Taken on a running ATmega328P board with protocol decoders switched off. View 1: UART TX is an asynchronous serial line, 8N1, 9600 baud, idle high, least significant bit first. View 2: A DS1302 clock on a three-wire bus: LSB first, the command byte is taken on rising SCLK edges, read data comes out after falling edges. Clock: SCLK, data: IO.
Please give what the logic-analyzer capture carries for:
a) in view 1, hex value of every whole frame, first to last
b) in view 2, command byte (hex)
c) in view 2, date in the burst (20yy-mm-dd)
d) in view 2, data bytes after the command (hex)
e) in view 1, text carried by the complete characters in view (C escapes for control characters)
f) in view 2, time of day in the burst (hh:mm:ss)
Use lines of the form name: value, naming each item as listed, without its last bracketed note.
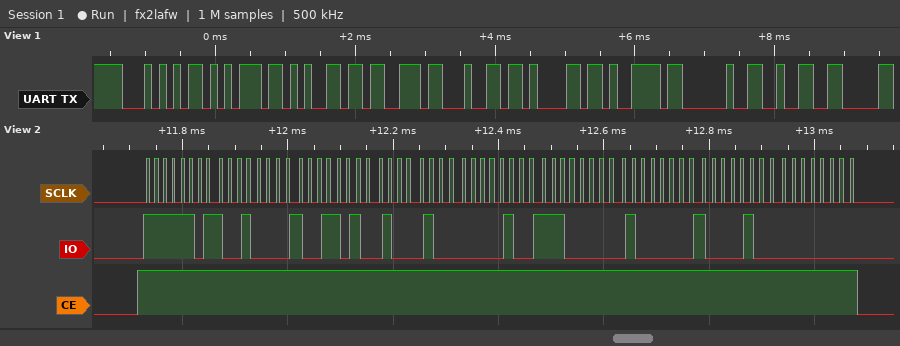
in view 1, hex value of every whole frame, first to last: 54 75 65 73 64 61 79 20 32
in view 2, command byte: 0xBF
in view 2, date in the burst: 2021-07-20
in view 2, data bytes after the command: 09 59 22 20 07 02 21 00
in view 1, text carried by the complete characters in view: "Tuesday 2"
in view 2, time of day in the burst: 22:59:09
